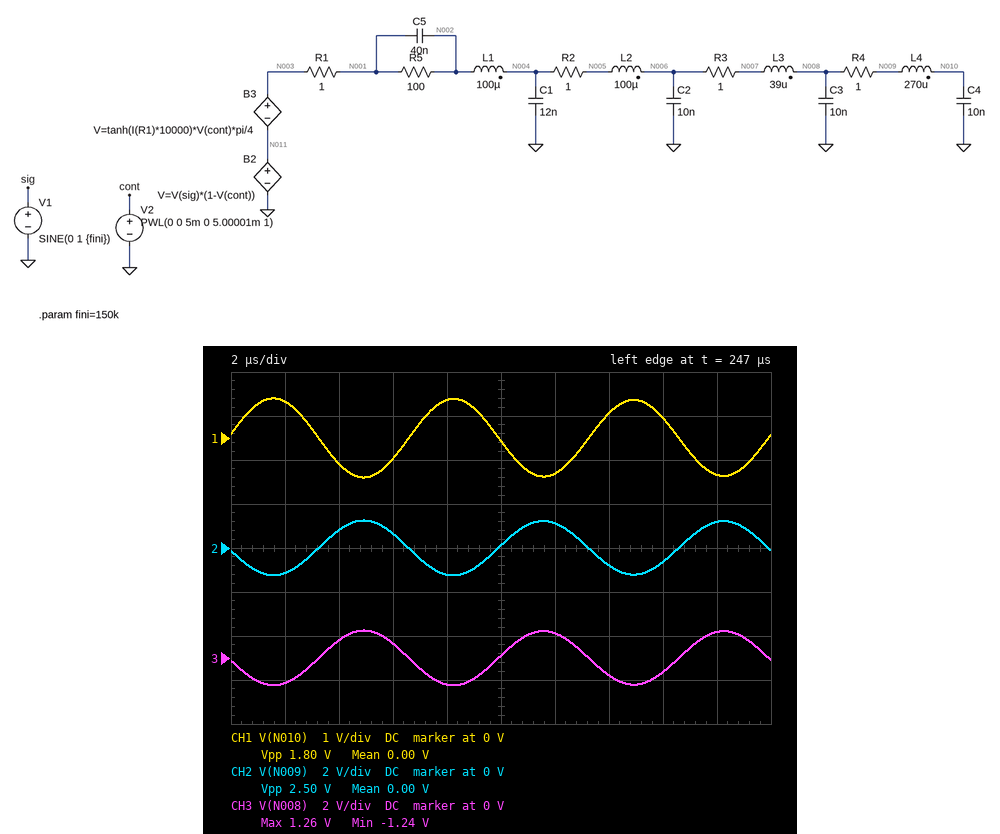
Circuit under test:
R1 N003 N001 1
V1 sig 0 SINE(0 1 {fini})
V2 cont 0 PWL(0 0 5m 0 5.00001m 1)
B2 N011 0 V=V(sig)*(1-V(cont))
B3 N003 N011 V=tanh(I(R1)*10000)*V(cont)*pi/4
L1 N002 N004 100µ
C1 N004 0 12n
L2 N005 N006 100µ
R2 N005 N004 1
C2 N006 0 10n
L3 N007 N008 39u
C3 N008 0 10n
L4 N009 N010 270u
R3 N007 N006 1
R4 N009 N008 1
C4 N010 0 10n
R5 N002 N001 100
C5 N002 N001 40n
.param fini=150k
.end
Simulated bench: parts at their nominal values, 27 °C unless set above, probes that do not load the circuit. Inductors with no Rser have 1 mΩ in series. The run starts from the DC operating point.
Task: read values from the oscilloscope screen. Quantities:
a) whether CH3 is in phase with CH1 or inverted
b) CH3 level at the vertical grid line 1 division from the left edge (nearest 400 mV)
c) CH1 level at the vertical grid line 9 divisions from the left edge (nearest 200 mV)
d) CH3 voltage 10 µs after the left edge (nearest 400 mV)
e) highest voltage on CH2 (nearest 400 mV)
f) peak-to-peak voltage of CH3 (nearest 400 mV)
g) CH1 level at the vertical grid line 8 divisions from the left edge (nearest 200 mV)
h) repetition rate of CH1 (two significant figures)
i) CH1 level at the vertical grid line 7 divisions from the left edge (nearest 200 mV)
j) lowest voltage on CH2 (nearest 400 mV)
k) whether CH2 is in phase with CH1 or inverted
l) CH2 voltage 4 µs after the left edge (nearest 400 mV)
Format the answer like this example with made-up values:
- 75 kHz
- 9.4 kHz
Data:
- inverted
- -1.2 V
- -800 mV
- 0 V
- 1.2 V
- 2.4 V
- 400 mV
- 150 kHz
- 600 mV
- -1.2 V
- inverted
- 800 mV
